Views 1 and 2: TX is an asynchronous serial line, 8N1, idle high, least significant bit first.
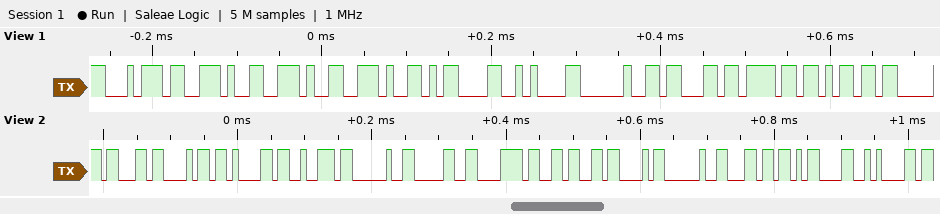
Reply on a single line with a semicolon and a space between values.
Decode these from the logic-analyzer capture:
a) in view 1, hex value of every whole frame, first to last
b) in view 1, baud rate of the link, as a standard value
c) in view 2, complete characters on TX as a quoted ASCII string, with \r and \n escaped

0x74 0x2E 0x2E 0x2E 0x0D 0x0A 0x20 0x63 0x6F 0x6D; 115200 baud; "char 0x6C l\r\n"
